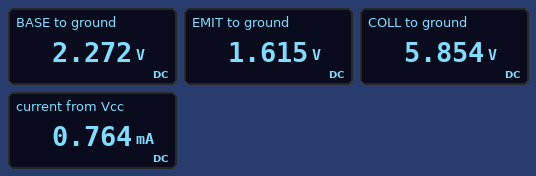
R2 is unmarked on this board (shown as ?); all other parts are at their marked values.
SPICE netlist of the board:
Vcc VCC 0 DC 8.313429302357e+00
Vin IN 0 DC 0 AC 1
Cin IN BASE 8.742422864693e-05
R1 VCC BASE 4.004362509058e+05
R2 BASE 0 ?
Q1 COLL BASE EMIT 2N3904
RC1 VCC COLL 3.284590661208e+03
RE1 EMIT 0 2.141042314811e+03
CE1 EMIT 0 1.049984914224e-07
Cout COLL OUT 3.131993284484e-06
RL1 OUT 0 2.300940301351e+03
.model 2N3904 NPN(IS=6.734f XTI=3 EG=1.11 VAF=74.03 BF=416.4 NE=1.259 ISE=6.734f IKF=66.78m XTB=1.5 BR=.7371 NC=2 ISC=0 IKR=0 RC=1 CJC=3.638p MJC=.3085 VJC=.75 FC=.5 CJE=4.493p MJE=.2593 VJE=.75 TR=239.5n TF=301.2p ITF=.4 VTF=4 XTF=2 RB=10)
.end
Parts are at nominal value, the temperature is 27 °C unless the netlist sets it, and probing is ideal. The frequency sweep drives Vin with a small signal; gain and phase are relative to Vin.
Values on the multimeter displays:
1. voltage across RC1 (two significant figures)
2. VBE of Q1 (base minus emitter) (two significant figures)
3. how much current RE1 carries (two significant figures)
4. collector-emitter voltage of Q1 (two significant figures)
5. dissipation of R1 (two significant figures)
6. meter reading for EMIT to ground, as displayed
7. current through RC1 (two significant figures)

2.5 V
660 mV
750 µA
4.2 V
91 µW
1.615 V
750 µA
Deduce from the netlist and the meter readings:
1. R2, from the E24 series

240 kΩ
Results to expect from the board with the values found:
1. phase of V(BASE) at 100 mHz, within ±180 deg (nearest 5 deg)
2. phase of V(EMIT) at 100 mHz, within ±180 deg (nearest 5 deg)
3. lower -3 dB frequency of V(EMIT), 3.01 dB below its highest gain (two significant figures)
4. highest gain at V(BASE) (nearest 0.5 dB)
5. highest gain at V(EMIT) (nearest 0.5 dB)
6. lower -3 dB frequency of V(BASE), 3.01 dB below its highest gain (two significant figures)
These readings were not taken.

10 deg
10 deg
18 mHz
0 dB
0 dB
18 mHz
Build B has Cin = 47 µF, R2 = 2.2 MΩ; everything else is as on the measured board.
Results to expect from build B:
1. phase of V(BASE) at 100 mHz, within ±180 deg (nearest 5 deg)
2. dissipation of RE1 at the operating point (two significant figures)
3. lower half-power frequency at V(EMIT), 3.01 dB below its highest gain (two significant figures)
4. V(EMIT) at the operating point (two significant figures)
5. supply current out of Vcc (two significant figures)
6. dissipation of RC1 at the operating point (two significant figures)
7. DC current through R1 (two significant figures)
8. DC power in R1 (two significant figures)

10 deg
4.1 mW
21 mHz
3.0 V
1.4 mA
6.3 mW
12 µA
54 µW
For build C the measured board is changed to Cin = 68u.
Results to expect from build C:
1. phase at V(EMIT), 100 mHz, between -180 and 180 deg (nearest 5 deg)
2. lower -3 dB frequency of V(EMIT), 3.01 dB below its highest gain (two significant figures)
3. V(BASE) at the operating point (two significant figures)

15 deg
23 mHz
2.3 V
